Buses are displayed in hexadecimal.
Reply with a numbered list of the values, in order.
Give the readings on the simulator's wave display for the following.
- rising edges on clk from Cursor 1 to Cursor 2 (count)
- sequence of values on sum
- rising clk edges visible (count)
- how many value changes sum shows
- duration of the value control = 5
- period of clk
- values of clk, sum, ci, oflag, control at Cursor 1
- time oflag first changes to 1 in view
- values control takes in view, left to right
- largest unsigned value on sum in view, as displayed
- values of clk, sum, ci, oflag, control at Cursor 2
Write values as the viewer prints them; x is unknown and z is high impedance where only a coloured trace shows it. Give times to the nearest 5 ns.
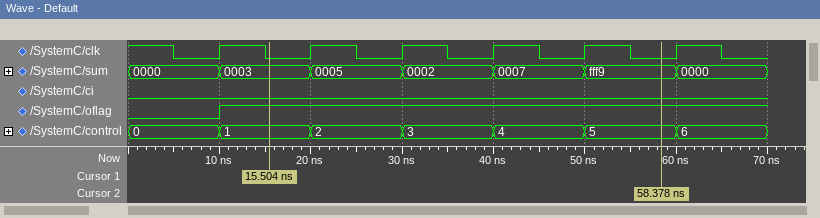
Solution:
1. 4
2. 0000, 0003, 0005, 0002, 0007, fff9, 0000
3. 6
4. 6
5. 10 ns
6. 10 ns
7. clk=0, sum=0003, ci=0, oflag=1, control=1
8. 10 ns
9. 0, 1, 2, 3, 4, 5, 6
10. fff9
11. clk=0, sum=fff9, ci=0, oflag=1, control=5
